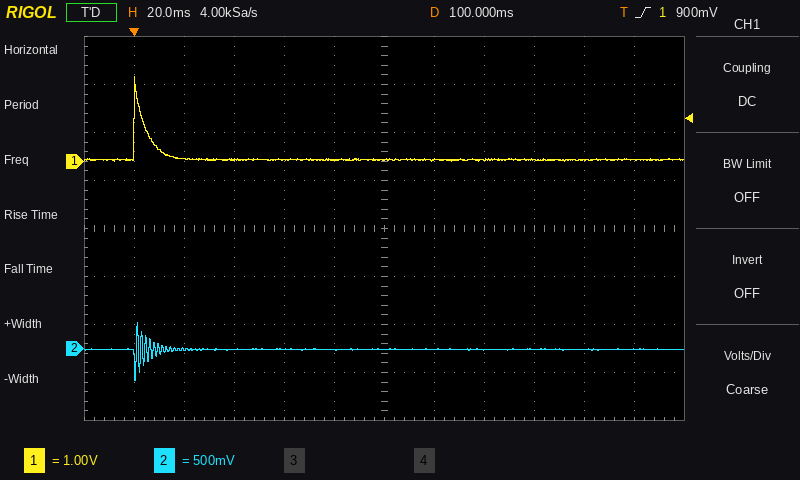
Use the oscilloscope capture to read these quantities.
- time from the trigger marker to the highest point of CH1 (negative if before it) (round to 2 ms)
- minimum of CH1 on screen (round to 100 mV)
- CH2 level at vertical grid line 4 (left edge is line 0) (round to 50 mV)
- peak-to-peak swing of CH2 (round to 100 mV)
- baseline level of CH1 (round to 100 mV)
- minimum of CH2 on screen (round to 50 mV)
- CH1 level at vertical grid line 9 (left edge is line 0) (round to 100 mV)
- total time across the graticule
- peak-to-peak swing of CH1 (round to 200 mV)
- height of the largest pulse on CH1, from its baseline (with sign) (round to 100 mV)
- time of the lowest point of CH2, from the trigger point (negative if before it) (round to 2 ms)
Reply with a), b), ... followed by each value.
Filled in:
a) 0 ms
b) 0.0 V
c) 0 mV
d) 600 mV
e) 0.0 V
f) -350 mV
g) 0.0 V
h) 240 ms
i) 1.8 V
j) +1.7 V
k) 0 ms
